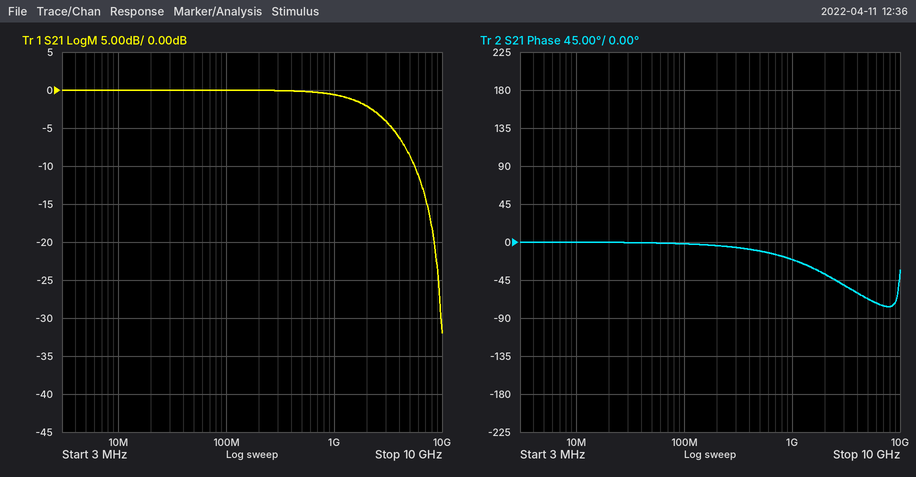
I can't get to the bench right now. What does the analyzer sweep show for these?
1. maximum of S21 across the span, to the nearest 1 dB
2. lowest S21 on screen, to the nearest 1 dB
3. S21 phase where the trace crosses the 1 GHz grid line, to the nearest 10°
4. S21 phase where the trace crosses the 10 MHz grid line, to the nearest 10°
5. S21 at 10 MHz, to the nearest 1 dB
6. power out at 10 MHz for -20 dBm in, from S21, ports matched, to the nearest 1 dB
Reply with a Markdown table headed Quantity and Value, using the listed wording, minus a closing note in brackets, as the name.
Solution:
| Quantity | Value |
|---|---|
| maximum of S21 across the span, to the nearest 1 dB | 0 dB |
| lowest S21 on screen, to the nearest 1 dB | -32 dB |
| S21 phase where the trace crosses the 1 GHz grid line, to the nearest 10° | -20° |
| S21 phase where the trace crosses the 10 MHz grid line, to the nearest 10° | 0° |
| S21 at 10 MHz, to the nearest 1 dB | 0 dB |
| power out at 10 MHz for -20 dBm in, from S21, ports matched, to the nearest 1 dB | -20 dBm |
